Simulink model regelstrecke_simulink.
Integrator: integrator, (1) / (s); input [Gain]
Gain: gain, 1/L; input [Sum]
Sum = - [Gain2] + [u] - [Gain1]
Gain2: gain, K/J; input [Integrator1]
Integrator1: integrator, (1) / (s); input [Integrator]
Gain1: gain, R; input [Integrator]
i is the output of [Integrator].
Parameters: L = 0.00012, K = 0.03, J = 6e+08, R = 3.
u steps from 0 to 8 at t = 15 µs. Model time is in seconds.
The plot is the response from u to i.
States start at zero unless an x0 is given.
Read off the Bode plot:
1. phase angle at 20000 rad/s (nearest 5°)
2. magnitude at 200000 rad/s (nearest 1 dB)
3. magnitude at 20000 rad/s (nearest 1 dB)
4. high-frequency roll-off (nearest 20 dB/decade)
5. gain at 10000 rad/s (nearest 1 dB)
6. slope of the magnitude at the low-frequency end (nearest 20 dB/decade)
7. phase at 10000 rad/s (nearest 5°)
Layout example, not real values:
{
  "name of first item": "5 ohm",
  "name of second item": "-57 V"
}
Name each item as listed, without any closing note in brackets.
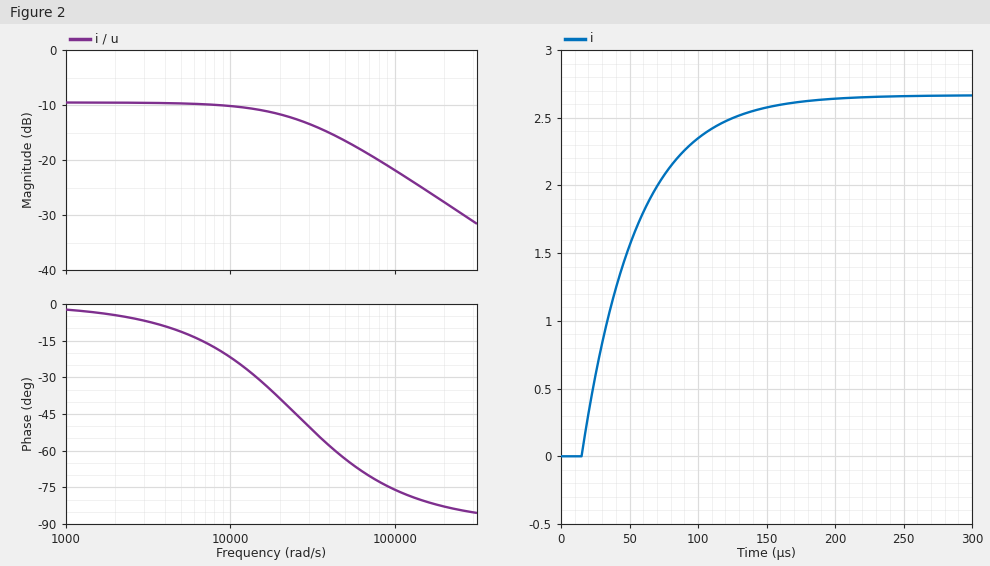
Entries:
{
  "phase angle at 20000 rad/s": "-40°",
  "magnitude at 200000 rad/s": "-28 dB",
  "magnitude at 20000 rad/s": "-12 dB",
  "high-frequency roll-off": "-20 dB/decade",
  "gain at 10000 rad/s": "-10 dB",
  "slope of the magnitude at the low-frequency end": "0 dB/decade",
  "phase at 10000 rad/s": "-20°"
}
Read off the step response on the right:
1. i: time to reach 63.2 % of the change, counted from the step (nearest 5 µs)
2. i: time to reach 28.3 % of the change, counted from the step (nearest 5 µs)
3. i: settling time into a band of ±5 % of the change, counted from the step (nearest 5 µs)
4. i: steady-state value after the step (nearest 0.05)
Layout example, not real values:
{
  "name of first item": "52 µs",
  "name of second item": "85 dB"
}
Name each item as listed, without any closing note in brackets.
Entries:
{
  "i: time to reach 63.2 % of the change, counted from the step": "40 µs",
  "i: time to reach 28.3 % of the change, counted from the step": "15 µs",
  "i: settling time into a band of ±5 % of the change, counted from the step": "120 µs",
  "i: steady-state value after the step": "2.65"
}
